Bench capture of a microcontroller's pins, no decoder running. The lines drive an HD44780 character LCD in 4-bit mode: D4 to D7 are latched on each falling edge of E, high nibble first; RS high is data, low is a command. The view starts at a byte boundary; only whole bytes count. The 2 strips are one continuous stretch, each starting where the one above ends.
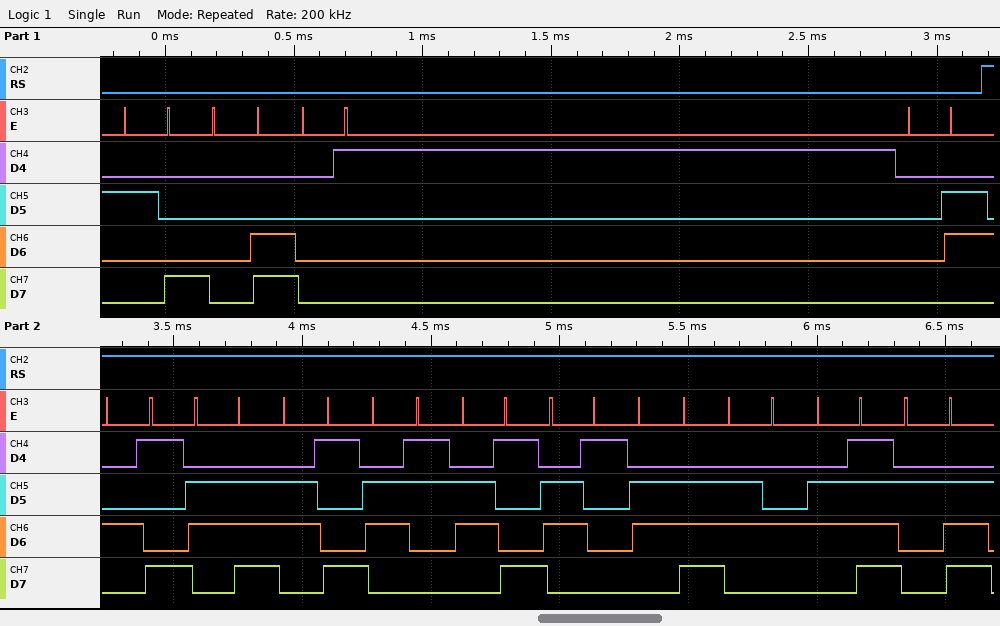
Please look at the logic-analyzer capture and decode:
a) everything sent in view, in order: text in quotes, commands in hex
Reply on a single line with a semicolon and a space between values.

0x28 0x0C 0x01 0x06 "Iniciando."
